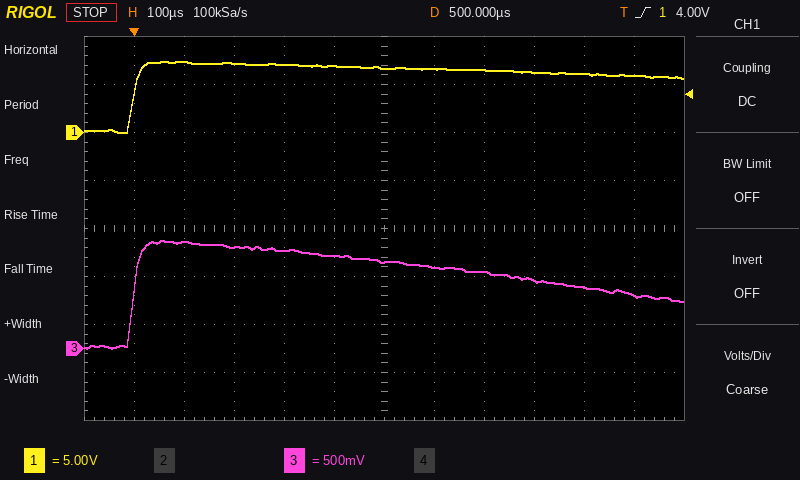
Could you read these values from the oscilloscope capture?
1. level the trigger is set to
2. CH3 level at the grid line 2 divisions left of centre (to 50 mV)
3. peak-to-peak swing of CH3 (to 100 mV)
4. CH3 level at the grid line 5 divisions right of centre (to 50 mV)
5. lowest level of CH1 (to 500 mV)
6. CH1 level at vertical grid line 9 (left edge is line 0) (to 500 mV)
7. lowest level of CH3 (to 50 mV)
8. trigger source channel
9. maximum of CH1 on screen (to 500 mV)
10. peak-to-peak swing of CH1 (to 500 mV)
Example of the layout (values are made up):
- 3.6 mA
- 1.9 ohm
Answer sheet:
- 4.00 V
- 1.00 V
- 1.10 V
- 550 mV
- 0.0 V
- 6.5 V
- 0 mV
- CH1
- 7.5 V
- 7.5 V
